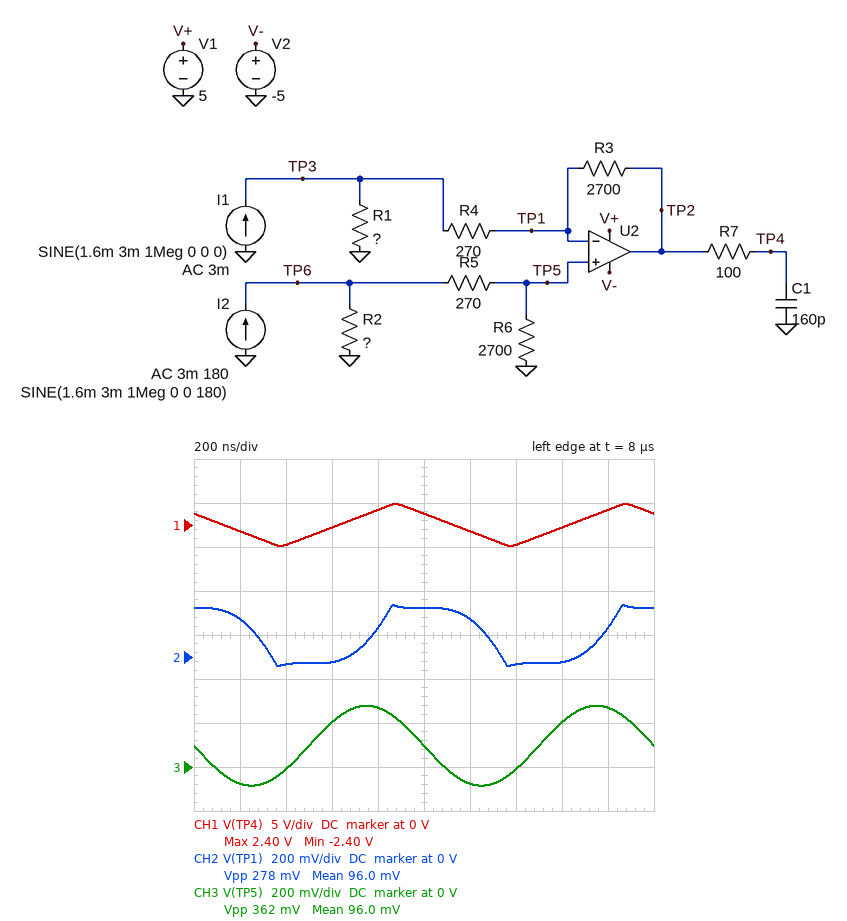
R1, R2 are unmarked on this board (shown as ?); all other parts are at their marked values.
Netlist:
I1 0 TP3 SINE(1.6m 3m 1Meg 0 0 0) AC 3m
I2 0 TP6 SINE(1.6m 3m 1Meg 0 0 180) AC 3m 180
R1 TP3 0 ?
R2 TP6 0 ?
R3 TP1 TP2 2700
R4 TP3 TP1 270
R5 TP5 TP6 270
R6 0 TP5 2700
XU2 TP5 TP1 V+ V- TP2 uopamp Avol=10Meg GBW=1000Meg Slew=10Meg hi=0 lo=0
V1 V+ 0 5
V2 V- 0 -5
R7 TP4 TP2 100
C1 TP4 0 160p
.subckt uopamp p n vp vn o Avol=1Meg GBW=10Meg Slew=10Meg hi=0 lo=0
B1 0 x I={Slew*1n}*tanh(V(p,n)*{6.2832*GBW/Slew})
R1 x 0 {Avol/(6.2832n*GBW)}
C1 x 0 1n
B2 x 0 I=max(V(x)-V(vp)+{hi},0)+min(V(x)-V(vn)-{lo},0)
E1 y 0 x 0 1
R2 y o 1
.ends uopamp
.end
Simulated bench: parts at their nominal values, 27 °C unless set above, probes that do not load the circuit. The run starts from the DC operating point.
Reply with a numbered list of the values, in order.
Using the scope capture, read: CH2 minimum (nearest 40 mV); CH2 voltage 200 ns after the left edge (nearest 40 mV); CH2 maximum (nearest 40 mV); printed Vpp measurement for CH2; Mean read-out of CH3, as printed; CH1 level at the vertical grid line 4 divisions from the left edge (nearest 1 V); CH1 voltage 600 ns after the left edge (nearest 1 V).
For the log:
1. -40 mV
2. 160 mV
3. 240 mV
4. 278 mV
5. 96.0 mV
6. 2 V
7. 0 V
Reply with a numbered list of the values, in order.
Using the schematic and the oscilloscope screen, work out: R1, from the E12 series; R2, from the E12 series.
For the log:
1. 68 Ω
2. 68 Ω
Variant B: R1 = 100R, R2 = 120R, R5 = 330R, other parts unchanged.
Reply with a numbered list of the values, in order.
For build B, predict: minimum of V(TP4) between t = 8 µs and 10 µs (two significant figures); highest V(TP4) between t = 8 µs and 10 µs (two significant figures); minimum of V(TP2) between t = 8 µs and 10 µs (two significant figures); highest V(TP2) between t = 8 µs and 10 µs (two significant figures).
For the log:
1. -2.2 V
2. 2.6 V
3. -2.3 V
4. 2.7 V
